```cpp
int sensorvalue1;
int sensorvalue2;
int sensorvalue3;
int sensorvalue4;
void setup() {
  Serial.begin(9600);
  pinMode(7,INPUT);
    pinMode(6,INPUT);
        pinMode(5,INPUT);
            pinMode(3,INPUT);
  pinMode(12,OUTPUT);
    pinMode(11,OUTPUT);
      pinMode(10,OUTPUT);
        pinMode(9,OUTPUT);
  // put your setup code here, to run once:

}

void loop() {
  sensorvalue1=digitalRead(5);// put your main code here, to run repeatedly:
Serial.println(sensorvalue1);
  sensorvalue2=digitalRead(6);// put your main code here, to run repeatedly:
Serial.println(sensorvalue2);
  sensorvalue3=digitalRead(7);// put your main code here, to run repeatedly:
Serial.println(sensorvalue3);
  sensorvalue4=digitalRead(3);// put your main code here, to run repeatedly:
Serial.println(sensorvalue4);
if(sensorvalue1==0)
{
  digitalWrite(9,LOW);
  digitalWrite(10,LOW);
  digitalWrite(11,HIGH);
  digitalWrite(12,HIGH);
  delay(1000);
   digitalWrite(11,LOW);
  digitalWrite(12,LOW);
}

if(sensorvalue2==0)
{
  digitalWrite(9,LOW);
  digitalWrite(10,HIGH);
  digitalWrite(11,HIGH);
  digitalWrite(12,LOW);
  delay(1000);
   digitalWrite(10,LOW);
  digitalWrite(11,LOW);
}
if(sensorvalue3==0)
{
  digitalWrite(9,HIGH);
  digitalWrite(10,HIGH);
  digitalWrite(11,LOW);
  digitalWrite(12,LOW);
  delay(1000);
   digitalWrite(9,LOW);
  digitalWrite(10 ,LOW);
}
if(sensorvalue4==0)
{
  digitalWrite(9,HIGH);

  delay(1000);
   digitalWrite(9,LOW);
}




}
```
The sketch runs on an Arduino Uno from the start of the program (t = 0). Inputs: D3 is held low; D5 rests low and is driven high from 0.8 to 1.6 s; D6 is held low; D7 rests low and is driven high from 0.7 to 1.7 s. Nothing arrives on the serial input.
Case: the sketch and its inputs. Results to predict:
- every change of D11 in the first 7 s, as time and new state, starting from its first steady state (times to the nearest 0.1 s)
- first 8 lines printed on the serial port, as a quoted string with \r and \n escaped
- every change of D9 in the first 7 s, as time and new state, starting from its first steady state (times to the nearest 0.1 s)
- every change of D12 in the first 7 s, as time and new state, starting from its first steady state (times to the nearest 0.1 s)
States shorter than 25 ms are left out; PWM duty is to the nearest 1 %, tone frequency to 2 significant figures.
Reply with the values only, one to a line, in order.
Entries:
0 s high; 2 s low; 4 s high; 6 s low
"0\r\n0\r\n0\r\n0\r\n0\r\n0\r\n0\r\n0\r\n"
0 s low; 2 s high; 4 s low; 6 s high
0 s high; 1 s low; 4 s high; 5 s low
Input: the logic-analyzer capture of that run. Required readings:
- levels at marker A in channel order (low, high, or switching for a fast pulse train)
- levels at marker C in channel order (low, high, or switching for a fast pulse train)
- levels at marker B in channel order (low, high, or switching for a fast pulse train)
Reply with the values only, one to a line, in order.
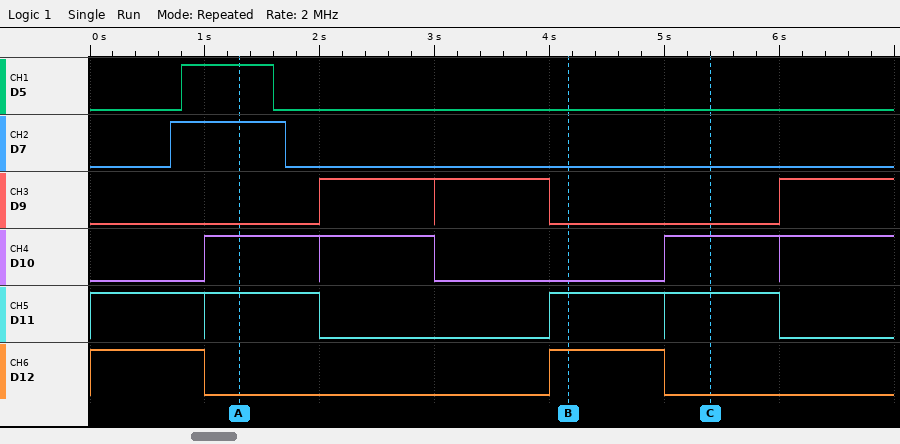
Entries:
D5 high, D7 high, D9 low, D10 high, D11 high, D12 low
D5 low, D7 low, D9 low, D10 high, D11 high, D12 low
D5 low, D7 low, D9 low, D10 low, D11 high, D12 high
